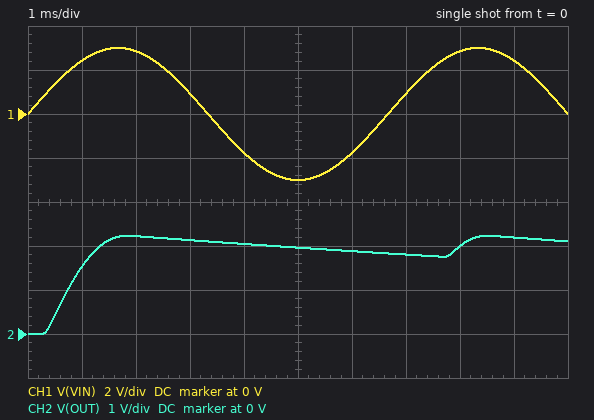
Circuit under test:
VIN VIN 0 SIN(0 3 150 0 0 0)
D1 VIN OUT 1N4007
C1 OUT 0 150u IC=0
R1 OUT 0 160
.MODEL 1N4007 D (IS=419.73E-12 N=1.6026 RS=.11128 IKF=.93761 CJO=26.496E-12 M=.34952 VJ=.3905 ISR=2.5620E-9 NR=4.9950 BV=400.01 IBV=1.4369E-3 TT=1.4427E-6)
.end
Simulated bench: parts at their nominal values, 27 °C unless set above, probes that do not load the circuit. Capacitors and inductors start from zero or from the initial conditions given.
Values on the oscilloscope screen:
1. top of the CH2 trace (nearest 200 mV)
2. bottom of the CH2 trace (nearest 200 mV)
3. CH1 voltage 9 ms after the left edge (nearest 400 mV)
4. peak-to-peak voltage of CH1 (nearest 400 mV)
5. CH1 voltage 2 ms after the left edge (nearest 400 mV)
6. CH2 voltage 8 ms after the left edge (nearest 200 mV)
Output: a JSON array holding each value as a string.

["2.2 V", "0 V", "2.4 V", "6.0 V", "2.8 V", "2.0 V"]
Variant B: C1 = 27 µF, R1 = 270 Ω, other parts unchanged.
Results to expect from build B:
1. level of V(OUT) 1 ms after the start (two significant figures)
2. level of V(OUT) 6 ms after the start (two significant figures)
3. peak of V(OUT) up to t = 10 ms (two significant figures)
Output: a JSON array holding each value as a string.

["1.6 V", "1.3 V", "2.3 V"]
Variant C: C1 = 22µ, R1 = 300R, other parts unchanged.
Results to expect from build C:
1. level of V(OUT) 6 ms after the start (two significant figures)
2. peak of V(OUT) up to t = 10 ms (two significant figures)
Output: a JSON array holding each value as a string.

["1.2 V", "2.3 V"]
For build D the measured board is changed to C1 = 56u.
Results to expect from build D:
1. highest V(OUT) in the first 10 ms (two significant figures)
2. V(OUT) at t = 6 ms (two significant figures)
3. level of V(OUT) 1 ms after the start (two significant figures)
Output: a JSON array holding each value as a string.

["2.3 V", "1.4 V", "1.6 V"]
